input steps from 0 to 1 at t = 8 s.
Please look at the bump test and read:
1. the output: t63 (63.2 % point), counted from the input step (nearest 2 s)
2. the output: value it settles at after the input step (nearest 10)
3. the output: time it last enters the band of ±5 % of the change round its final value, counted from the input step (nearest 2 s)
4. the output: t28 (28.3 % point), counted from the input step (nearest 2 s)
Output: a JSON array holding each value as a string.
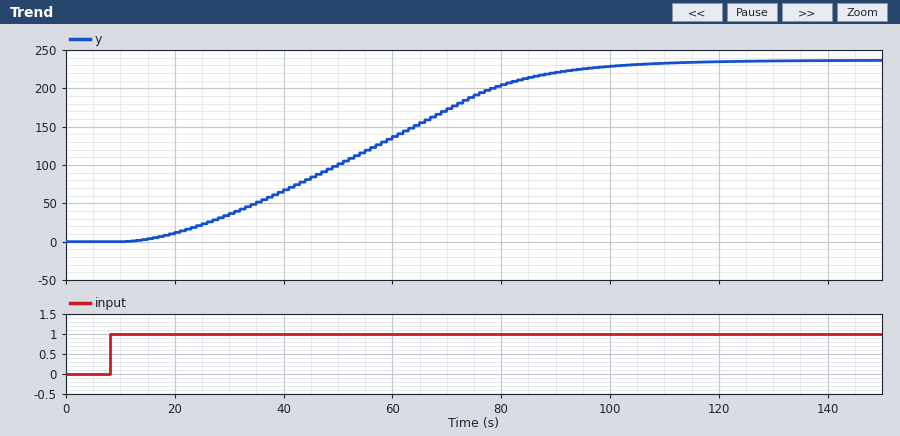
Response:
["56 s", "240", "86 s", "32 s"]
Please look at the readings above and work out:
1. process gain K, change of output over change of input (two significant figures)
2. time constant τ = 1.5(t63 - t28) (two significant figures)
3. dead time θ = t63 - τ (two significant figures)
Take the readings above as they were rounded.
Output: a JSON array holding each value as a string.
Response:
["240", "36 s", "20 s"]
